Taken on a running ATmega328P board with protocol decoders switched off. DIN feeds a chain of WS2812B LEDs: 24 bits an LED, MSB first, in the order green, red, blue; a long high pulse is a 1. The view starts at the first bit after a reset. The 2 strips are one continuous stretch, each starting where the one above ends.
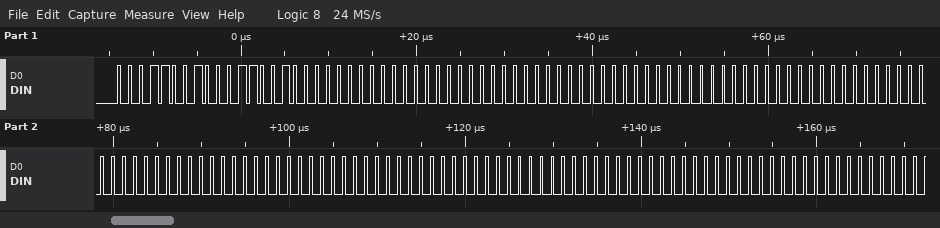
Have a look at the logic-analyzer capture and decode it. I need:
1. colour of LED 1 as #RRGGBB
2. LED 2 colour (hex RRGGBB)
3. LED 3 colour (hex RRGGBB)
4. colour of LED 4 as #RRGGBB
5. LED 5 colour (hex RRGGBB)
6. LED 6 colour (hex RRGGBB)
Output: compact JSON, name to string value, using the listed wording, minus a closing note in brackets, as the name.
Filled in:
{"colour of LED 1 as #RRGGBB": "#191900", "LED 2 colour": "#000000", "LED 3 colour": "#000000", "colour of LED 4 as #RRGGBB": "#000000", "LED 5 colour": "#000000", "LED 6 colour": "#000000"}
